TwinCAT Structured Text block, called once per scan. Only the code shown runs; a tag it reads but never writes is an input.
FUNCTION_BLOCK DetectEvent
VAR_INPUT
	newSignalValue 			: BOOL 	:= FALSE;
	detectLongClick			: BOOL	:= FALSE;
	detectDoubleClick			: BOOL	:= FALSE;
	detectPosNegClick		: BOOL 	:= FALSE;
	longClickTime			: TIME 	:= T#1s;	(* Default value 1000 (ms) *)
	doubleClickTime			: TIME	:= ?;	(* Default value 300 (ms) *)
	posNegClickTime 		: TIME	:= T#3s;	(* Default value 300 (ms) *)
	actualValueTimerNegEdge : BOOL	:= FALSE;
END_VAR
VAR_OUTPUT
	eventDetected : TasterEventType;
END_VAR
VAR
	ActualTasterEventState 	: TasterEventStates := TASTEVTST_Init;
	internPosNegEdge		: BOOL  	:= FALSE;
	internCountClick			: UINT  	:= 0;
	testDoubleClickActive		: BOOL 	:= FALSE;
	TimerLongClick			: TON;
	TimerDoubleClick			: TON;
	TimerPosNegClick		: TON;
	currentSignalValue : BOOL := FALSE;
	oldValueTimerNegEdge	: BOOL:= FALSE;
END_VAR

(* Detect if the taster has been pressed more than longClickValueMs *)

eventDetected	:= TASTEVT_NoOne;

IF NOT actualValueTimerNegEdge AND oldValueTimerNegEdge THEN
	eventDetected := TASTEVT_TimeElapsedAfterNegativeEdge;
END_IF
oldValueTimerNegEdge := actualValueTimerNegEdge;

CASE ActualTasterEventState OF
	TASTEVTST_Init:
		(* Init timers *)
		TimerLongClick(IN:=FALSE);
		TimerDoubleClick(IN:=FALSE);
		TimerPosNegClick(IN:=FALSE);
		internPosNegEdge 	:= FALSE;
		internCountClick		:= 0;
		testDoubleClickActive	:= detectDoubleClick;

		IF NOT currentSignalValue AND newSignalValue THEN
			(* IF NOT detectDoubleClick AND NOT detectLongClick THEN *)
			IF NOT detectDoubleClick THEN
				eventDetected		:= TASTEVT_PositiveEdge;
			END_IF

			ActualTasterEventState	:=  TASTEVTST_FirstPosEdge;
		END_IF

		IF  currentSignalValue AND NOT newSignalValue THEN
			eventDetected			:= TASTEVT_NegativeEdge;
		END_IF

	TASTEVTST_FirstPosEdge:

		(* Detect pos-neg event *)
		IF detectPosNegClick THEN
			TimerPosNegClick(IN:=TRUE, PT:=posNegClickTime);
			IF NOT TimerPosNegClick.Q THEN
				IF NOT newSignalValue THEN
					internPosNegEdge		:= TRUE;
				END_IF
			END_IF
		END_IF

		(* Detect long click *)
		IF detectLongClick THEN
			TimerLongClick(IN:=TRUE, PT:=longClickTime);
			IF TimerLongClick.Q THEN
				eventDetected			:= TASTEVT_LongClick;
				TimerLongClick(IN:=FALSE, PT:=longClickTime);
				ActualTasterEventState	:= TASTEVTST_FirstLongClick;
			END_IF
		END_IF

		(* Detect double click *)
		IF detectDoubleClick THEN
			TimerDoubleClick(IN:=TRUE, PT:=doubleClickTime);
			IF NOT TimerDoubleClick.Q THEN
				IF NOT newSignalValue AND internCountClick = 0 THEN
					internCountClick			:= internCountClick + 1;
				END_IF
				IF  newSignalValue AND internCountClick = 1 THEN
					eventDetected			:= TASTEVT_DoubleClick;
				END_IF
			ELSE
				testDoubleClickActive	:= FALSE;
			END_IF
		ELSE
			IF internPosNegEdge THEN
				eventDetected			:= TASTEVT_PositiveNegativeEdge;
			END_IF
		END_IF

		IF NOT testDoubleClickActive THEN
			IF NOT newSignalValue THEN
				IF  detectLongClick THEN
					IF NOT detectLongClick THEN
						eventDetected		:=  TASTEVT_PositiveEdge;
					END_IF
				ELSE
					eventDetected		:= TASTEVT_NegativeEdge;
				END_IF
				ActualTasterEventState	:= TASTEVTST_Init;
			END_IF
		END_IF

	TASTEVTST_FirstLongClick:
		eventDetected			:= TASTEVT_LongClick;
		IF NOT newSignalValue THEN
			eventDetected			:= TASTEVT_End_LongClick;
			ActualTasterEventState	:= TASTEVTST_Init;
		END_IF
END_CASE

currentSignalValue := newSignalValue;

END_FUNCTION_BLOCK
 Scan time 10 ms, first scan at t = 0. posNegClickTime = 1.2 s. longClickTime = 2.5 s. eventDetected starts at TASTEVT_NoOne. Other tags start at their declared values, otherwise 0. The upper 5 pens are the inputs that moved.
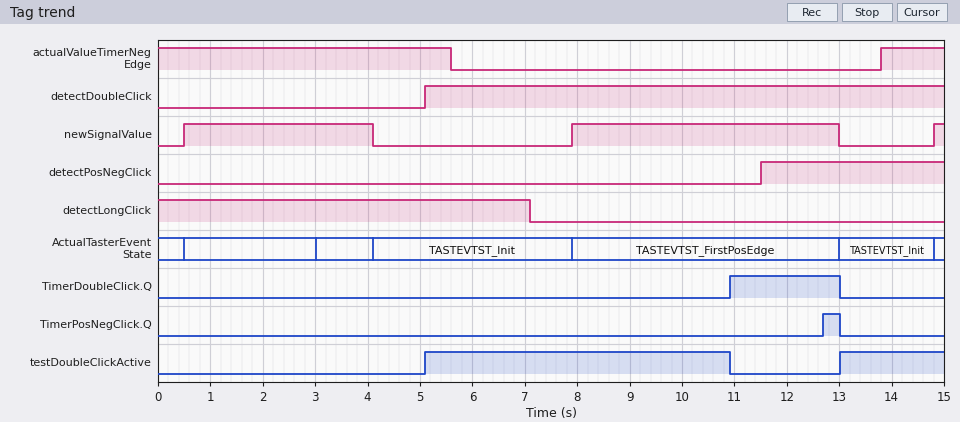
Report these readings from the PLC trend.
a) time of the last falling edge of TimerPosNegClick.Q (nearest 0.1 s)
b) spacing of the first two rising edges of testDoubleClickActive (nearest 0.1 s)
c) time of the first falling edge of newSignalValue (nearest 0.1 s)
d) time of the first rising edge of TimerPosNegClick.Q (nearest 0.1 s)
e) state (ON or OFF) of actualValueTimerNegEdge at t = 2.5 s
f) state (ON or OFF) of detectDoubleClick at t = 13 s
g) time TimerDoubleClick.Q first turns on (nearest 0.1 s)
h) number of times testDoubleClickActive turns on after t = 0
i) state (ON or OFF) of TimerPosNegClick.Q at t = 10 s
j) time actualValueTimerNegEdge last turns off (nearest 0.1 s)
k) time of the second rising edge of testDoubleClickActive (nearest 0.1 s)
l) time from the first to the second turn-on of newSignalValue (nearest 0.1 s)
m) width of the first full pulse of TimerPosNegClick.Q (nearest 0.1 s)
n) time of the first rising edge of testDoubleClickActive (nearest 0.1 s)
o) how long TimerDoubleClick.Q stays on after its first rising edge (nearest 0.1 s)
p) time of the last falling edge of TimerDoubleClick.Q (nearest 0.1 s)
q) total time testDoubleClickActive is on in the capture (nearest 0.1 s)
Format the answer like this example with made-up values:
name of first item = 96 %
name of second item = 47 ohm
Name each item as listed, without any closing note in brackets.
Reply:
time of the last falling edge of TimerPosNegClick.Q = 13.0 s
spacing of the first two rising edges of testDoubleClickActive = 7.9 s
time of the first falling edge of newSignalValue = 4.1 s
time of the first rising edge of TimerPosNegClick.Q = 12.7 s
state (ON or OFF) of actualValueTimerNegEdge at t = 2.5 s = ON
state (ON or OFF) of detectDoubleClick at t = 13 s = ON
time TimerDoubleClick.Q first turns on = 10.9 s
number of times testDoubleClickActive turns on after t = 0 = 2
state (ON or OFF) of TimerPosNegClick.Q at t = 10 s = OFF
time actualValueTimerNegEdge last turns off = 5.6 s
time of the second rising edge of testDoubleClickActive = 13.0 s
time from the first to the second turn-on of newSignalValue = 7.4 s
width of the first full pulse of TimerPosNegClick.Q = 0.3 s
time of the first rising edge of testDoubleClickActive = 5.1 s
how long TimerDoubleClick.Q stays on after its first rising edge = 2.1 s
time of the last falling edge of TimerDoubleClick.Q = 13.0 s
total time testDoubleClickActive is on in the capture = 7.8 s
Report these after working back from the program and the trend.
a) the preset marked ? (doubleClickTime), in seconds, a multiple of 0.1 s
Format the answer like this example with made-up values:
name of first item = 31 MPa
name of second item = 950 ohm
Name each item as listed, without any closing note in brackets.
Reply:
the preset marked ? (doubleClickTime), in seconds, a multiple of 0.1 s = 3.0 s
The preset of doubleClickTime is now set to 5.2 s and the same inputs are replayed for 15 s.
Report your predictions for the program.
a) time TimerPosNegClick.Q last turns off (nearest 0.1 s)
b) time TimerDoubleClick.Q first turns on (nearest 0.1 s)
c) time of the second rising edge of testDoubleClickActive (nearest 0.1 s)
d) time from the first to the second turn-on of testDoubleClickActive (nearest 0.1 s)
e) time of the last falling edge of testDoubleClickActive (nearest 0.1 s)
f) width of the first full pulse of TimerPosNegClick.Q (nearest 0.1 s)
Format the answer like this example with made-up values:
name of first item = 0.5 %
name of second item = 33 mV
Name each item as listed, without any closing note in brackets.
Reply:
time TimerPosNegClick.Q last turns off = 13.1 s
time TimerDoubleClick.Q first turns on = 13.1 s
time of the second rising edge of testDoubleClickActive = 13.1 s
time from the first to the second turn-on of testDoubleClickActive = 8.0 s
time of the last falling edge of testDoubleClickActive = 13.1 s
width of the first full pulse of TimerPosNegClick.Q = 0.4 s
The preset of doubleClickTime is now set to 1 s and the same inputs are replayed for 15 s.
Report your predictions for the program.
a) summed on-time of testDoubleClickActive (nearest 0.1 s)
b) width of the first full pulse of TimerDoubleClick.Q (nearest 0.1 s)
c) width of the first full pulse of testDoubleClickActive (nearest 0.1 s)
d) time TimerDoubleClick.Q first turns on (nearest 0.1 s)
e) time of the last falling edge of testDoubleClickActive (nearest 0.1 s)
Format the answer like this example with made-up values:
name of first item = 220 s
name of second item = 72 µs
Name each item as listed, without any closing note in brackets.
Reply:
summed on-time of testDoubleClickActive = 5.8 s
width of the first full pulse of TimerDoubleClick.Q = 4.1 s
width of the first full pulse of testDoubleClickActive = 3.8 s
time TimerDoubleClick.Q first turns on = 8.9 s
time of the last falling edge of testDoubleClickActive = 8.9 s
